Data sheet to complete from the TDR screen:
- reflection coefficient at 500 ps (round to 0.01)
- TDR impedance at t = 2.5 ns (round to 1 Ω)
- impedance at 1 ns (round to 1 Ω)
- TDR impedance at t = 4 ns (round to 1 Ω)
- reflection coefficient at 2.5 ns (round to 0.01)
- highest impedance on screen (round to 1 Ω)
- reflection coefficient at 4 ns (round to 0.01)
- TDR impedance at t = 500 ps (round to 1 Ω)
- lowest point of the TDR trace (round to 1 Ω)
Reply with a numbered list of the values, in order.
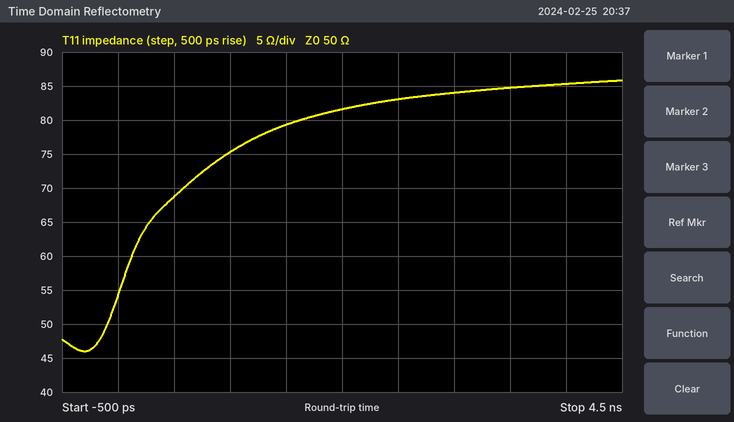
1. +0.16
2. 83 Ω
3. 75 Ω
4. 85 Ω
5. +0.25
6. 86 Ω
7. +0.26
8. 69 Ω
9. 46 Ω
